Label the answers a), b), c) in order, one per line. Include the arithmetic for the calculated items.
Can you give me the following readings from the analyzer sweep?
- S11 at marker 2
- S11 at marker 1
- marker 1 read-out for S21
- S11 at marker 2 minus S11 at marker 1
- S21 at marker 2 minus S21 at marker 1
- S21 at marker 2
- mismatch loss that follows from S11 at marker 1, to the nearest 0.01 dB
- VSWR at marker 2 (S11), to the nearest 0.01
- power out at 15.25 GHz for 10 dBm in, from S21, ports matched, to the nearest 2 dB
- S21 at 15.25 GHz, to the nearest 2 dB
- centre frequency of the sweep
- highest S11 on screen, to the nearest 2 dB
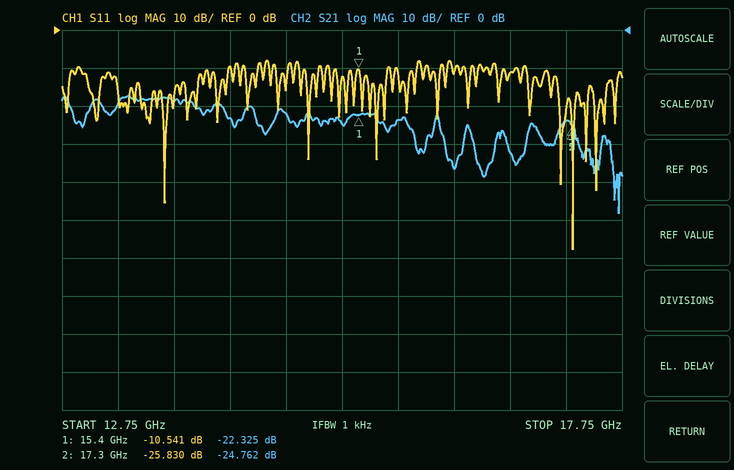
a) -25.830 dB
b) -10.541 dB
c) -22.325 dB
d) -25.83 − (-10.541) = -15.289 dB
e) -24.762 − (-22.325) = -2.437 dB
f) -24.762 dB
g) −10 log10(1 − 10^(-10.541/10)) ≈ 0.40 dB
h) (1 + 0.0511)/(1 − 0.0511) ≈ 1.11
i) 10 dBm + (-24 dB) = -14 dBm
j) -24 dB
k) 15.25 GHz
l) -8 dB
